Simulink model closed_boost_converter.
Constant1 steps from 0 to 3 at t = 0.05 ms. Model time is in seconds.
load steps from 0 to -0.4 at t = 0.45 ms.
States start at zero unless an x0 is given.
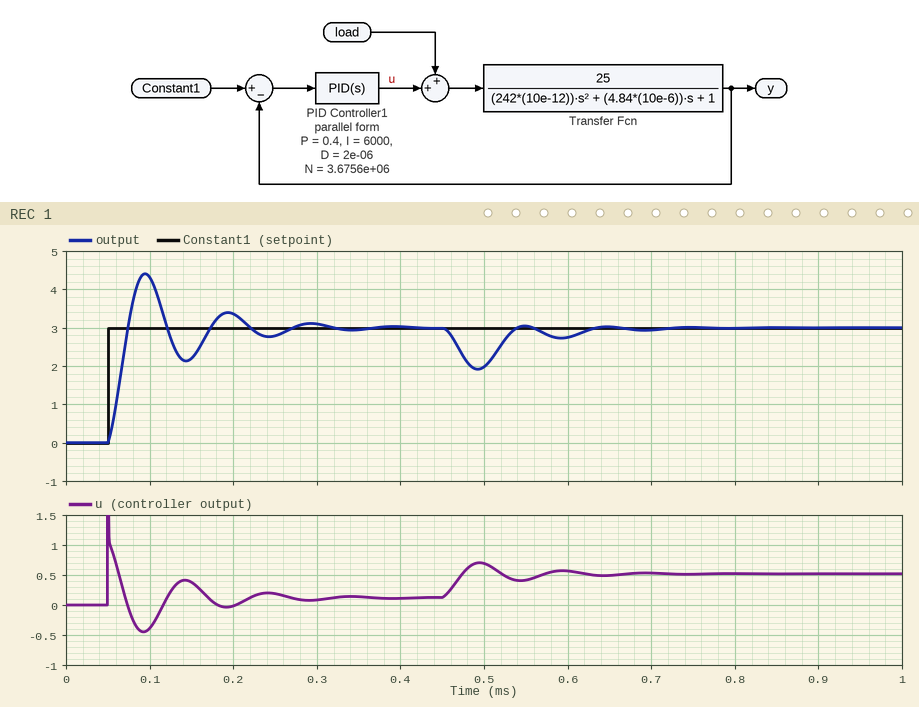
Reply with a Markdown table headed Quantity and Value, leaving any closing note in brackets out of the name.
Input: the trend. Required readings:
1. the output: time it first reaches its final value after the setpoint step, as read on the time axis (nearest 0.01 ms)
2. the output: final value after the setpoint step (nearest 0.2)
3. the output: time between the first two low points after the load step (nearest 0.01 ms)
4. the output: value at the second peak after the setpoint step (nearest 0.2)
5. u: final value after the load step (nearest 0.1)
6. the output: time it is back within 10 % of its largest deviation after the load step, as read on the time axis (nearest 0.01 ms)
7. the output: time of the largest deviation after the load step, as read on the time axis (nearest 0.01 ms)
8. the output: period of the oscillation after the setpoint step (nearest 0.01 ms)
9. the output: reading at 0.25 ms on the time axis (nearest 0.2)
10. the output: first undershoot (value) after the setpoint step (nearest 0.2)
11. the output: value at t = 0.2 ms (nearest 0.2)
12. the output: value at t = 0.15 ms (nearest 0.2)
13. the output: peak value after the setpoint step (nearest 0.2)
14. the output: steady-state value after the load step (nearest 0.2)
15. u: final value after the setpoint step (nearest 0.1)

| Quantity | Value |
|---|---|
| the output: time it first reaches its final value after the setpoint step, as read on the time axis | 0.07 ms |
| the output: final value after the setpoint step | 3.0 |
| the output: time between the first two low points after the load step | 0.10 ms |
| the output: value at the second peak after the setpoint step | 3.4 |
| u: final value after the load step | 0.5 |
| the output: time it is back within 10 % of its largest deviation after the load step, as read on the time axis | 0.62 ms |
| the output: time of the largest deviation after the load step, as read on the time axis | 0.49 ms |
| the output: period of the oscillation after the setpoint step | 0.10 ms |
| the output: reading at 0.25 ms on the time axis | 2.8 |
| the output: first undershoot (value) after the setpoint step | 2.2 |
| the output: value at t = 0.2 ms | 3.4 |
| the output: value at t = 0.15 ms | 2.2 |
| the output: peak value after the setpoint step | 4.4 |
| the output: steady-state value after the load step | 3.0 |
| u: final value after the setpoint step | 0.1 |
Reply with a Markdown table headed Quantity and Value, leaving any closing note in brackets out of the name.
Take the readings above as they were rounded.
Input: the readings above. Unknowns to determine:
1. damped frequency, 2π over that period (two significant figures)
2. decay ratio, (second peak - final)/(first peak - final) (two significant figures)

| Quantity | Value |
|---|---|
| damped frequency, 2π over that period | 63 rad/ms |
| decay ratio, (second peak - final)/(first peak - final) | 0.29 |
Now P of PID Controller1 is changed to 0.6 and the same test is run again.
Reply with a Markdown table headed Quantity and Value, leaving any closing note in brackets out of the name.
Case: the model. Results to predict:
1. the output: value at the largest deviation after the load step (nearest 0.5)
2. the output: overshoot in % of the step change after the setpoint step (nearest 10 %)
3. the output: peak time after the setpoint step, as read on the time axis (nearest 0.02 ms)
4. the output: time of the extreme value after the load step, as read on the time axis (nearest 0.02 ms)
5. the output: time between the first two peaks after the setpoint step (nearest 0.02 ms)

| Quantity | Value |
|---|---|
| the output: value at the largest deviation after the load step | 2.0 |
| the output: overshoot in % of the step change after the setpoint step | 50 % |
| the output: peak time after the setpoint step, as read on the time axis | 0.08 ms |
| the output: time of the extreme value after the load step, as read on the time axis | 0.48 ms |
| the output: time between the first two peaks after the setpoint step | 0.08 ms |
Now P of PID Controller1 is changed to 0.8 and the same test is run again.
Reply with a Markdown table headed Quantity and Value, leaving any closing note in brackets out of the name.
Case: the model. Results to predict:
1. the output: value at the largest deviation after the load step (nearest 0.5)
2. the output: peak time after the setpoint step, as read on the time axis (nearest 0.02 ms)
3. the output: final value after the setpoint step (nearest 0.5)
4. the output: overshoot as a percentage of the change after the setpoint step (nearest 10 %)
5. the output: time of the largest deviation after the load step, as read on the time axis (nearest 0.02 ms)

| Quantity | Value |
|---|---|
| the output: value at the largest deviation after the load step | 2.5 |
| the output: peak time after the setpoint step, as read on the time axis | 0.08 ms |
| the output: final value after the setpoint step | 3.0 |
| the output: overshoot as a percentage of the change after the setpoint step | 50 % |
| the output: time of the largest deviation after the load step, as read on the time axis | 0.48 ms |
